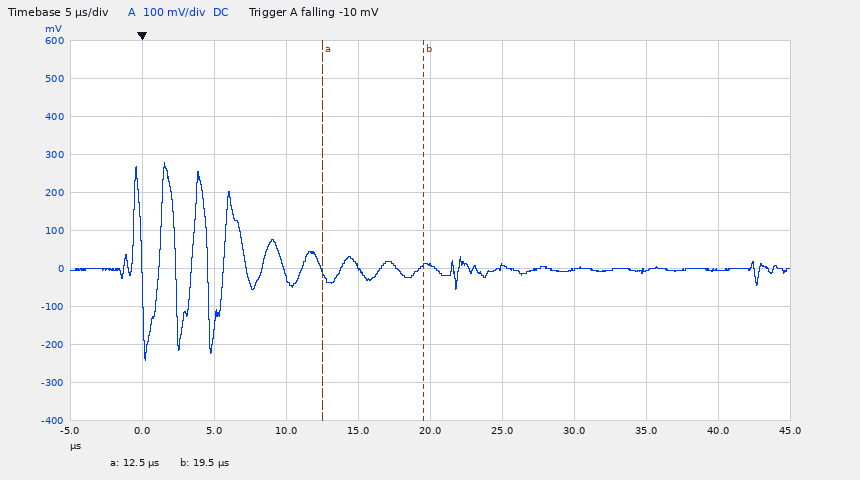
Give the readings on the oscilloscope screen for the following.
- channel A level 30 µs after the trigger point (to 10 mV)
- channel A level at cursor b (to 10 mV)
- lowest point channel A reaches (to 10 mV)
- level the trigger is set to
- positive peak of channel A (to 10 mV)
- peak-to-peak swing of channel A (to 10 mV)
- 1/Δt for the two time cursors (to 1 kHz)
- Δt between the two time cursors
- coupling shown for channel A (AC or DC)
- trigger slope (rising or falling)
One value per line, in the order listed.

0 mV
10 mV
-240 mV
-10 mV
280 mV
520 mV
143 kHz
7.0 µs
DC
falling
